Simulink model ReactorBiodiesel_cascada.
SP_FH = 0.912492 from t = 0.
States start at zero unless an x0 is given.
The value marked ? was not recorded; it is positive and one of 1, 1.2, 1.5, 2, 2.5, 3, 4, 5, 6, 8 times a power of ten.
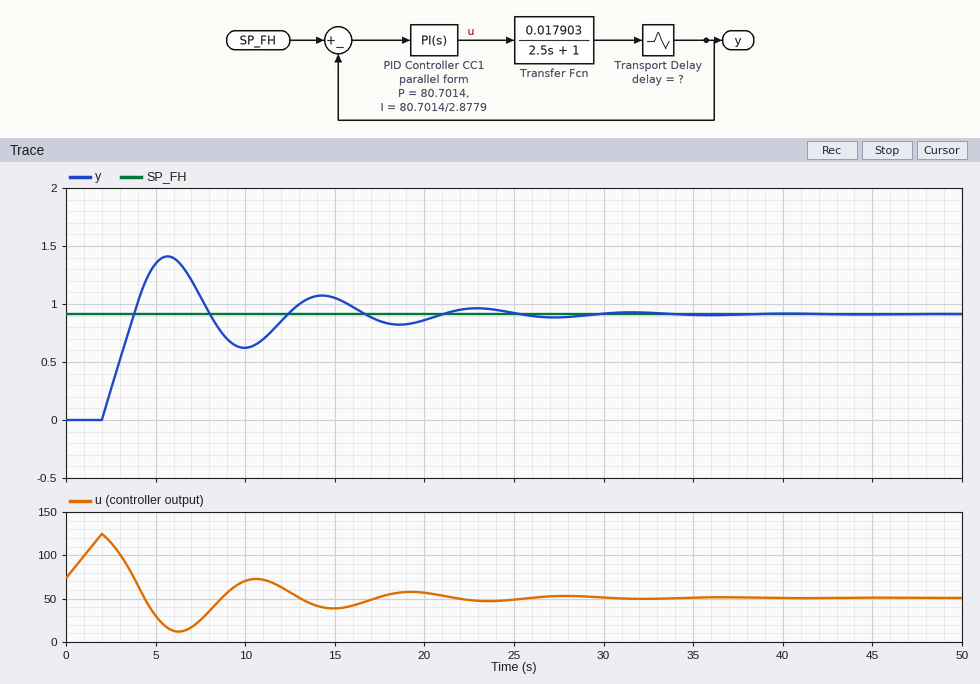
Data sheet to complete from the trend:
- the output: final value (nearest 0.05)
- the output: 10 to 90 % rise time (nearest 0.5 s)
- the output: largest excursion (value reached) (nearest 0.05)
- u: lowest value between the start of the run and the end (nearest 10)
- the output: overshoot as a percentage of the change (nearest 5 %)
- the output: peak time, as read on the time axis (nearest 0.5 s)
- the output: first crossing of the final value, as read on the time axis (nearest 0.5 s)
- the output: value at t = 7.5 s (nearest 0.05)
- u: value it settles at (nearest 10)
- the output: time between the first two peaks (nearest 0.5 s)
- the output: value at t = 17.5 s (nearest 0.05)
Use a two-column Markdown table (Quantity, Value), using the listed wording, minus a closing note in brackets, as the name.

| Quantity | Value |
|---|---|
| the output: final value | 0.90 |
| the output: 10 to 90 % rise time | 1.5 s |
| the output: largest excursion (value reached) | 1.40 |
| u: lowest value between the start of the run and the end | 10 |
| the output: overshoot as a percentage of the change | 55 % |
| the output: peak time, as read on the time axis | 5.5 s |
| the output: first crossing of the final value, as read on the time axis | 4.0 s |
| the output: value at t = 7.5 s | 1.05 |
| u: value it settles at | 50 |
| the output: time between the first two peaks | 8.5 s |
| the output: value at t = 17.5 s | 0.85 |
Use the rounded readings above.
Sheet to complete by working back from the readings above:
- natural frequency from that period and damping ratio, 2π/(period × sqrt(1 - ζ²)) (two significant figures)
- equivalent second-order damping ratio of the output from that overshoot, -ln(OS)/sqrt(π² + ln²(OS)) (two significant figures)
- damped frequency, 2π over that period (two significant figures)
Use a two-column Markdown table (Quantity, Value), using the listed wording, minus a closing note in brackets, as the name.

| Quantity | Value |
|---|---|
| natural frequency from that period and damping ratio, 2π/(period × sqrt(1 - ζ²)) | 0.75 rad/s |
| equivalent second-order damping ratio of the output from that overshoot, -ln(OS)/sqrt(π² + ln²(OS)) | 0.19 |
| damped frequency, 2π over that period | 0.74 rad/s |
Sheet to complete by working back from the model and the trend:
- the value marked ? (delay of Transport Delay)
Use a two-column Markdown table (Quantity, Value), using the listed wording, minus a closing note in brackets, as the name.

| Quantity | Value |
|---|---|
| the value marked ? | 2 |
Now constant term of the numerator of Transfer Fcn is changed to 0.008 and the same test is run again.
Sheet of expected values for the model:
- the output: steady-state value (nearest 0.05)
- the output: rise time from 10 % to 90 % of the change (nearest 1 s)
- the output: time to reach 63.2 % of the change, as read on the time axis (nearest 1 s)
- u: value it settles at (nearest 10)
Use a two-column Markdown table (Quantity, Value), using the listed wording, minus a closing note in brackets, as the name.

| Quantity | Value |
|---|---|
| the output: steady-state value | 0.90 |
| the output: rise time from 10 % to 90 % of the change | 4 s |
| the output: time to reach 63.2 % of the change, as read on the time axis | 5 s |
| u: value it settles at | 110 |
